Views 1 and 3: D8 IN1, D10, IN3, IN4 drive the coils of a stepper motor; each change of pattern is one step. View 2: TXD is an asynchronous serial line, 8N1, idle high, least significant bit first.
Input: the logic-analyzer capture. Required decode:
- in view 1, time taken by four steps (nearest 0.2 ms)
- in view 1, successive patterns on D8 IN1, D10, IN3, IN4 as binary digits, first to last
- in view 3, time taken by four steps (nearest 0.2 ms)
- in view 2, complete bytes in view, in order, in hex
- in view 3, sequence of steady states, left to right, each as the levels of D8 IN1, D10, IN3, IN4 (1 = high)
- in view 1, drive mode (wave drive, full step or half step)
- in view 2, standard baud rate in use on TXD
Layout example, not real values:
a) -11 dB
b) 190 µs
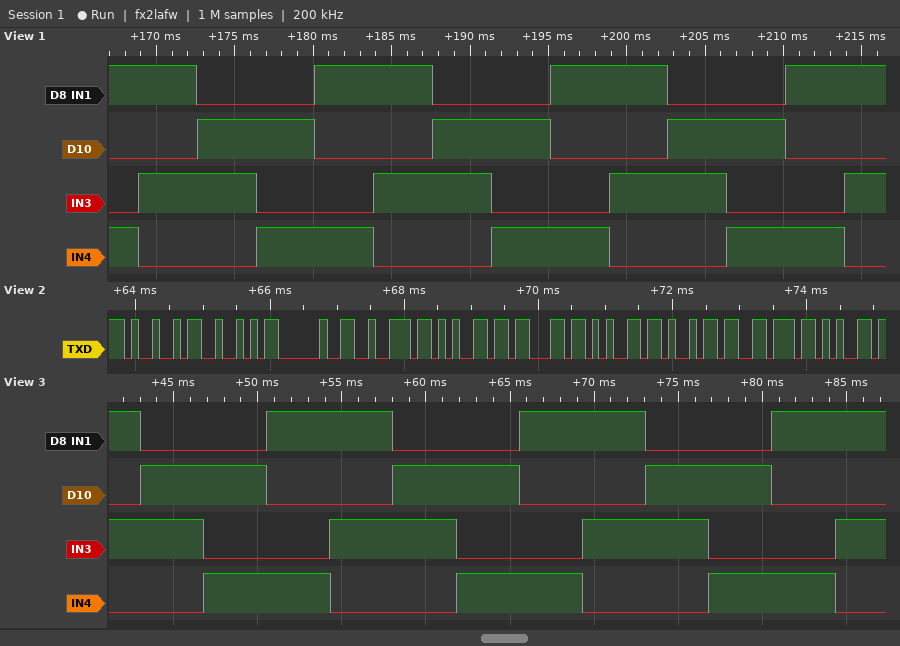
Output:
a) 15.0 ms
b) 1001 1010 0110 0101 1001 1010 0110 0101 1001 1010 0110 0101 1001 1010
c) 15.0 ms
d) 49 52 20 72 65 63 65 69 76 65
e) 1010 0110 0101 1001 1010 0110 0101 1001 1010 0110 0101 1001 1010
f) full step
g) 9600 baud
